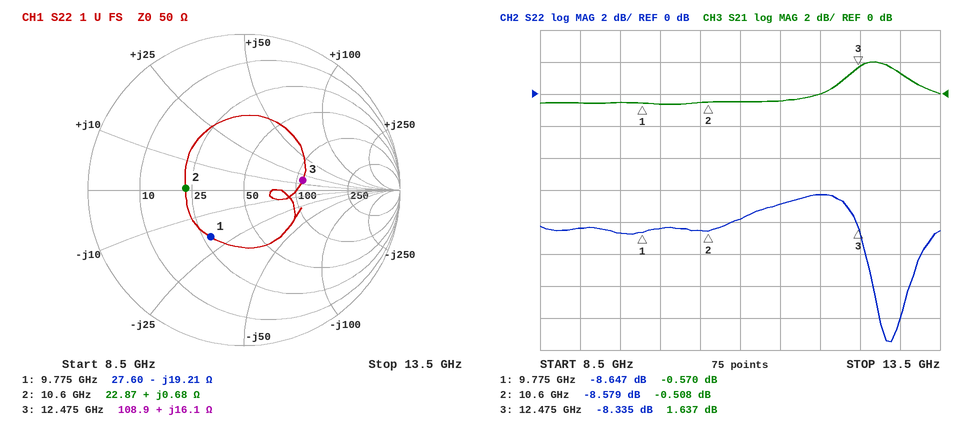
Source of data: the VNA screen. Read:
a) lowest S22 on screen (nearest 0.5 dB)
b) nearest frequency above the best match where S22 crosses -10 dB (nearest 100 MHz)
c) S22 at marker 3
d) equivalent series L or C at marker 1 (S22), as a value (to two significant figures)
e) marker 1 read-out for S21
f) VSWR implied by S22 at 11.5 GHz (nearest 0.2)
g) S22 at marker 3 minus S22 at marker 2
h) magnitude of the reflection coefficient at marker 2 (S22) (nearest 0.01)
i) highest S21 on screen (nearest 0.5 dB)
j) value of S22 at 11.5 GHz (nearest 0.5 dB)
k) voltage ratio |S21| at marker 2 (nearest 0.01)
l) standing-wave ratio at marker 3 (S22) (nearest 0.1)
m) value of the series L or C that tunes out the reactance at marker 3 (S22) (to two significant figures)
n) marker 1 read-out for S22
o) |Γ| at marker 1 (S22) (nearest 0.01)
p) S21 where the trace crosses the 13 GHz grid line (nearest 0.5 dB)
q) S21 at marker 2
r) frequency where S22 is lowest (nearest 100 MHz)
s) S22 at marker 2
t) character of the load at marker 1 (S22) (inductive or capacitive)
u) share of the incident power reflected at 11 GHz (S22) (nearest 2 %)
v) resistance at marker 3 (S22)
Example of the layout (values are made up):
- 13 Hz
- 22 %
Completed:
- -15.5 dB
- 13.3 GHz
- -8.335 dB
- 850 fF
- -0.570 dB
- 2.6
- 0.244 dB
- 0.37
- 2.0 dB
- -7.0 dB
- 0.94
- 2.2
- 790 fF
- -8.647 dB
- 0.37
- 1.5 dB
- -0.508 dB
- 12.9 GHz
- -8.579 dB
- capacitive
- 16 %
- 108.9 Ω
